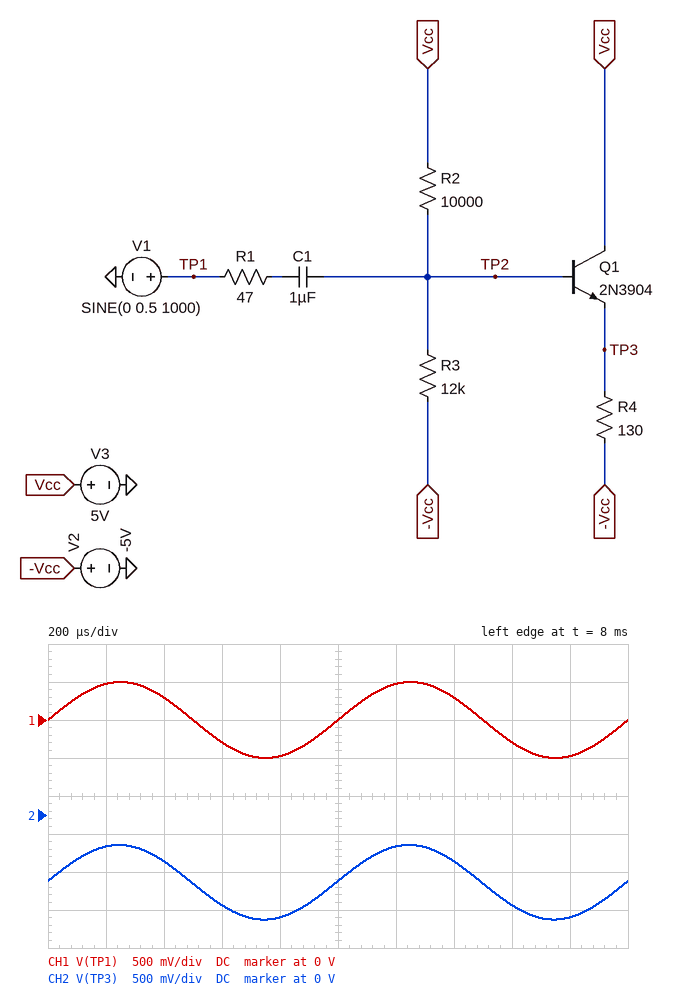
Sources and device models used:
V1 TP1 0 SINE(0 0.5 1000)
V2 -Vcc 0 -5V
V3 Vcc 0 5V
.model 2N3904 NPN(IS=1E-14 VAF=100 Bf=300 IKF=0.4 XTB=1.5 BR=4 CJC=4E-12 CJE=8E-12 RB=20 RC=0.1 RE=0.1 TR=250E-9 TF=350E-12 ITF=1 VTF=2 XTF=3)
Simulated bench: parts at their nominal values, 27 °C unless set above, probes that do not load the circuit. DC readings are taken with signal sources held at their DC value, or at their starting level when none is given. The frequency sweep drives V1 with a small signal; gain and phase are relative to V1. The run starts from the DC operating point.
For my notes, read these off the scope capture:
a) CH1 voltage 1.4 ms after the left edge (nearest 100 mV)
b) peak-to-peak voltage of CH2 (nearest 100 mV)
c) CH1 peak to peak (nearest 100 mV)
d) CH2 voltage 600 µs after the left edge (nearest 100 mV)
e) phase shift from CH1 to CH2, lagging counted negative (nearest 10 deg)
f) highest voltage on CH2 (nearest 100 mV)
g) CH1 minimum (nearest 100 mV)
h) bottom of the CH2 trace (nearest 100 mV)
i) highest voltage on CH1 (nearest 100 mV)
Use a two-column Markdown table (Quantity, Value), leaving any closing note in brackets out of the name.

| Quantity | Value |
|---|---|
| CH1 voltage 1.4 ms after the left edge | 300 mV |
| peak-to-peak voltage of CH2 | 1.0 V |
| CH1 peak to peak | 1.0 V |
| CH2 voltage 600 µs after the left edge | -1.2 V |
| phase shift from CH1 to CH2, lagging counted negative | 0 deg |
| highest voltage on CH2 | -400 mV |
| CH1 minimum | -500 mV |
| bottom of the CH2 trace | -1.4 V |
| highest voltage on CH1 | 500 mV |
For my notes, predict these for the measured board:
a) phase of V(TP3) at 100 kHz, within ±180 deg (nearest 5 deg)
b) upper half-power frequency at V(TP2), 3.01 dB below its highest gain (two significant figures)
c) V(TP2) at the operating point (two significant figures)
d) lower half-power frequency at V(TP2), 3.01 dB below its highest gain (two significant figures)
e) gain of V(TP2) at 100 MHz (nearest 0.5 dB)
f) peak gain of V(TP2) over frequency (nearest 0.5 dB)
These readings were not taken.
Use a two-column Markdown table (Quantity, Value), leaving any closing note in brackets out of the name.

| Quantity | Value |
|---|---|
| phase of V(TP3) at 100 kHz, within ±180 deg | 0 deg |
| upper half-power frequency at V(TP2), 3.01 dB below its highest gain | 730 MHz |
| V(TP2) at the operating point | -130 mV |
| lower half-power frequency at V(TP2), 3.01 dB below its highest gain | 33 Hz |
| gain of V(TP2) at 100 MHz | -0.5 dB |
| peak gain of V(TP2) over frequency | 0 dB |
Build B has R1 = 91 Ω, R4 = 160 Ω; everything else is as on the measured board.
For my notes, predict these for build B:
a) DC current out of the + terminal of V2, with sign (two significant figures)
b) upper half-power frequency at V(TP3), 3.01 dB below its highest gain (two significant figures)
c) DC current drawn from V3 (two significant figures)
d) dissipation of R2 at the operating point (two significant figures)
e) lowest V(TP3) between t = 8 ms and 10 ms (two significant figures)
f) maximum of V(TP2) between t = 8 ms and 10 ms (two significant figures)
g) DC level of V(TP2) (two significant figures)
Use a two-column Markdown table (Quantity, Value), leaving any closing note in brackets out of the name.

| Quantity | Value |
|---|---|
| DC current out of the + terminal of V2, with sign | -27 mA |
| upper half-power frequency at V(TP3), 3.01 dB below its highest gain | 300 MHz |
| DC current drawn from V3 | 27 mA |
| dissipation of R2 at the operating point | 2.5 mW |
| lowest V(TP3) between t = 8 ms and 10 ms | -1.3 V |
| maximum of V(TP2) between t = 8 ms and 10 ms | 460 mV |
| DC level of V(TP2) | -30 mV |
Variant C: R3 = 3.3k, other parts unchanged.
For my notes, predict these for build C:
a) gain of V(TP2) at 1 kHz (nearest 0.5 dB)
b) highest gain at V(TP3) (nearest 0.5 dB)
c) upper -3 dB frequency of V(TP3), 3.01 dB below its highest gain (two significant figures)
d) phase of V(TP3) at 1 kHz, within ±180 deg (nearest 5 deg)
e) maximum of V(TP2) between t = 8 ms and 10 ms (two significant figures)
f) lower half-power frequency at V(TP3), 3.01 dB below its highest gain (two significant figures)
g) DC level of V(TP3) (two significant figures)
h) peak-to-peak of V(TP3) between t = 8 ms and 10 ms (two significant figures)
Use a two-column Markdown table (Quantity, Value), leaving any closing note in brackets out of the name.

| Quantity | Value |
|---|---|
| gain of V(TP2) at 1 kHz | 0 dB |
| highest gain at V(TP3) | -0.5 dB |
| upper -3 dB frequency of V(TP3), 3.01 dB below its highest gain | 490 MHz |
| phase of V(TP3) at 1 kHz, within ±180 deg | 5 deg |
| maximum of V(TP2) between t = 8 ms and 10 ms | -2.1 V |
| lower half-power frequency at V(TP3), 3.01 dB below its highest gain | 67 Hz |
| DC level of V(TP3) | -3.3 V |
| peak-to-peak of V(TP3) between t = 8 ms and 10 ms | 960 mV |
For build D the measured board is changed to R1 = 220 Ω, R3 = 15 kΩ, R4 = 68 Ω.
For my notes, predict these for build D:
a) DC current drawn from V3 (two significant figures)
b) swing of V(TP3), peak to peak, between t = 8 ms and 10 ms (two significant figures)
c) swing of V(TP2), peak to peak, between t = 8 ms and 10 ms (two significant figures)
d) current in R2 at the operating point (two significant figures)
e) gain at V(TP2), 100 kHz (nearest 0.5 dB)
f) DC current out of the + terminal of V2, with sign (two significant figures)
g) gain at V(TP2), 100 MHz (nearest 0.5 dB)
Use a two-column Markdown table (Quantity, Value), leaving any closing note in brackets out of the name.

| Quantity | Value |
|---|---|
| DC current drawn from V3 | 59 mA |
| swing of V(TP3), peak to peak, between t = 8 ms and 10 ms | 940 mV |
| swing of V(TP2), peak to peak, between t = 8 ms and 10 ms | 950 mV |
| current in R2 at the operating point | 530 µA |
| gain at V(TP2), 100 kHz | -0.5 dB |
| DC current out of the + terminal of V2, with sign | -59 mA |
| gain at V(TP2), 100 MHz | -4.0 dB |
